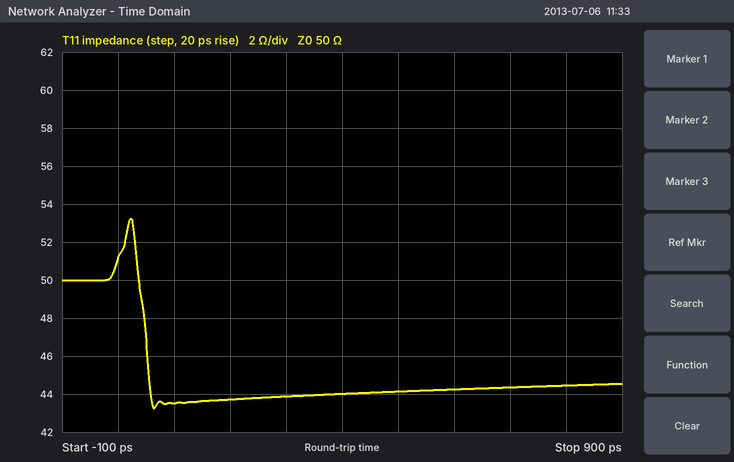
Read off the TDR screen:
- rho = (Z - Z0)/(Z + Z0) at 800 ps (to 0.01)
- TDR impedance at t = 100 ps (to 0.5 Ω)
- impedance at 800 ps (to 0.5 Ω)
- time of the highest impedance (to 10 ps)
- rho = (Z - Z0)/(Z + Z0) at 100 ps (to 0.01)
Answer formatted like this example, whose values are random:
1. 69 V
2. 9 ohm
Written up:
1. -0.06
2. 43.5 Ω
3. 44.5 Ω
4. 20 ps
5. -0.07
